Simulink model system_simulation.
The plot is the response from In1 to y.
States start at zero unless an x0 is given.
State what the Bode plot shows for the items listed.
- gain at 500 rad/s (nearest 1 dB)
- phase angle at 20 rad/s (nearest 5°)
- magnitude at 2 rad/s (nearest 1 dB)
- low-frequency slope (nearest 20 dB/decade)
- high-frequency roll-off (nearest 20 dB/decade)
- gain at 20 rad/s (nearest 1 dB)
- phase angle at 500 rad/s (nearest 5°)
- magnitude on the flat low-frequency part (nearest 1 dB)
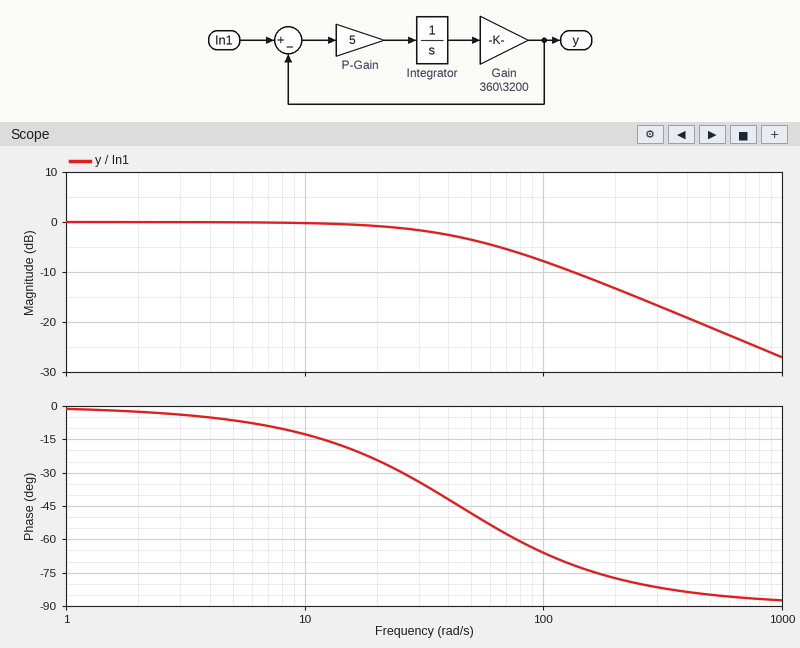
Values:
-21 dB
-25°
0 dB
0 dB/decade
-20 dB/decade
-1 dB
-85°
0 dB
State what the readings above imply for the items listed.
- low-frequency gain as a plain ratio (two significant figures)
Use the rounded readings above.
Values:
1.0
